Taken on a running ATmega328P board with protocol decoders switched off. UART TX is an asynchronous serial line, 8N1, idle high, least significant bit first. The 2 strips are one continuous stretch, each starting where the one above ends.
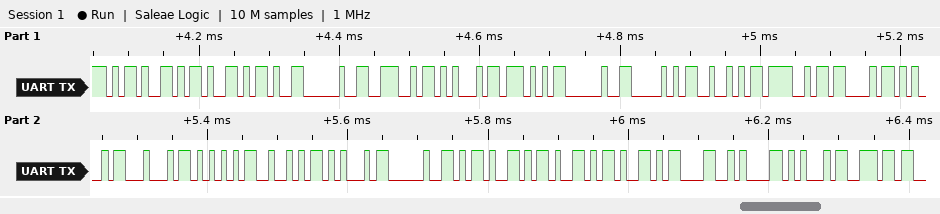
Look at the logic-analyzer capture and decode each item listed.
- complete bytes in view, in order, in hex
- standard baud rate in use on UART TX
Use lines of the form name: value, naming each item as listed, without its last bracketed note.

complete bytes in view, in order, in hex: 2D 2D 2D 20 4E 45 57 20 50 52 4F 43 45 44 55 52 45 20 2D 2D 2D 0D 0A 45 6E
standard baud rate in use on UART TX: 115200 baud
